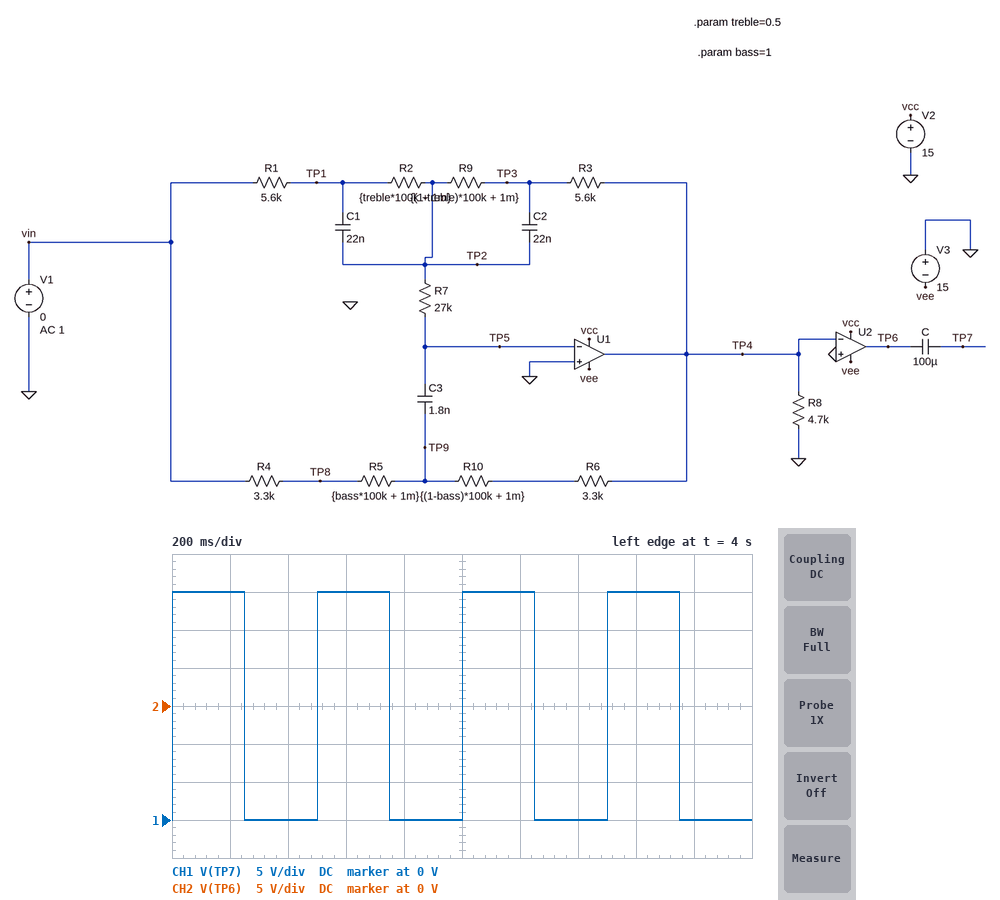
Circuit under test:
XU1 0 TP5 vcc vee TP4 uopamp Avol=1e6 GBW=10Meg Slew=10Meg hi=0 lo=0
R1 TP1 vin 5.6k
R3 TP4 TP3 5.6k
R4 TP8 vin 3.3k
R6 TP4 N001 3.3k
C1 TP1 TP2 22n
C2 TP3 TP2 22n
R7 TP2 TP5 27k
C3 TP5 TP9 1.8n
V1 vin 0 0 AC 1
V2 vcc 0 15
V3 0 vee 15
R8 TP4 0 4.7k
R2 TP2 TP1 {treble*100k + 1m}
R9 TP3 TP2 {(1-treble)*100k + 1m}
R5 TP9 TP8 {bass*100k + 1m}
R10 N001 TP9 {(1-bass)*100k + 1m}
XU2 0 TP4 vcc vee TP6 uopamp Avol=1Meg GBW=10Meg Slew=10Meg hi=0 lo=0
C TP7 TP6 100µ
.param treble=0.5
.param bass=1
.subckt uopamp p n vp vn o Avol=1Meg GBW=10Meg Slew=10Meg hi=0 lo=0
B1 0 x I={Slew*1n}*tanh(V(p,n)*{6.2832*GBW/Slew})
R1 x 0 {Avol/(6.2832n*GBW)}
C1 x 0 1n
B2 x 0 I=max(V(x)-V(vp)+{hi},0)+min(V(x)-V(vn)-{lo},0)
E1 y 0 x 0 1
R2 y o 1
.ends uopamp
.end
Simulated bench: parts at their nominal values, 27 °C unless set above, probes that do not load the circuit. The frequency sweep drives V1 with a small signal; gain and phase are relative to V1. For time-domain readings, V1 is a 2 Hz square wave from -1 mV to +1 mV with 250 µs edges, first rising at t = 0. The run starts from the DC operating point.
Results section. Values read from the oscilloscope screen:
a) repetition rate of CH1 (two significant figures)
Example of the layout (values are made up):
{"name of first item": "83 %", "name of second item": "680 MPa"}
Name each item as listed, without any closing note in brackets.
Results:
{"repetition rate of CH1": "2.0 Hz"}
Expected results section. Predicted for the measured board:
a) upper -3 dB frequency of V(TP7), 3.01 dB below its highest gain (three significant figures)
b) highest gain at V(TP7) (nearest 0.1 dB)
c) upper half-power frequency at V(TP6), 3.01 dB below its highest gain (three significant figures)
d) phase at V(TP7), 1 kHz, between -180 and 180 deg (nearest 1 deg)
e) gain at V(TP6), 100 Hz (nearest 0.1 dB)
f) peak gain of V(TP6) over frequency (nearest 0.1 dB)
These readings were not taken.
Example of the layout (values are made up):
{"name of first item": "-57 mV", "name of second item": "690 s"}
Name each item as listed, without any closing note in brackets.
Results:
{"upper -3 dB frequency of V(TP7), 3.01 dB below its highest gain": "9.99 Hz", "highest gain at V(TP7)": "120.0 dB", "upper half-power frequency at V(TP6), 3.01 dB below its highest gain": "9.99 Hz", "phase at V(TP7), 1 kHz, between -180 and 180 deg": "-119 deg", "gain at V(TP6), 100 Hz": "99.7 dB", "peak gain of V(TP6) over frequency": "120.0 dB"}
